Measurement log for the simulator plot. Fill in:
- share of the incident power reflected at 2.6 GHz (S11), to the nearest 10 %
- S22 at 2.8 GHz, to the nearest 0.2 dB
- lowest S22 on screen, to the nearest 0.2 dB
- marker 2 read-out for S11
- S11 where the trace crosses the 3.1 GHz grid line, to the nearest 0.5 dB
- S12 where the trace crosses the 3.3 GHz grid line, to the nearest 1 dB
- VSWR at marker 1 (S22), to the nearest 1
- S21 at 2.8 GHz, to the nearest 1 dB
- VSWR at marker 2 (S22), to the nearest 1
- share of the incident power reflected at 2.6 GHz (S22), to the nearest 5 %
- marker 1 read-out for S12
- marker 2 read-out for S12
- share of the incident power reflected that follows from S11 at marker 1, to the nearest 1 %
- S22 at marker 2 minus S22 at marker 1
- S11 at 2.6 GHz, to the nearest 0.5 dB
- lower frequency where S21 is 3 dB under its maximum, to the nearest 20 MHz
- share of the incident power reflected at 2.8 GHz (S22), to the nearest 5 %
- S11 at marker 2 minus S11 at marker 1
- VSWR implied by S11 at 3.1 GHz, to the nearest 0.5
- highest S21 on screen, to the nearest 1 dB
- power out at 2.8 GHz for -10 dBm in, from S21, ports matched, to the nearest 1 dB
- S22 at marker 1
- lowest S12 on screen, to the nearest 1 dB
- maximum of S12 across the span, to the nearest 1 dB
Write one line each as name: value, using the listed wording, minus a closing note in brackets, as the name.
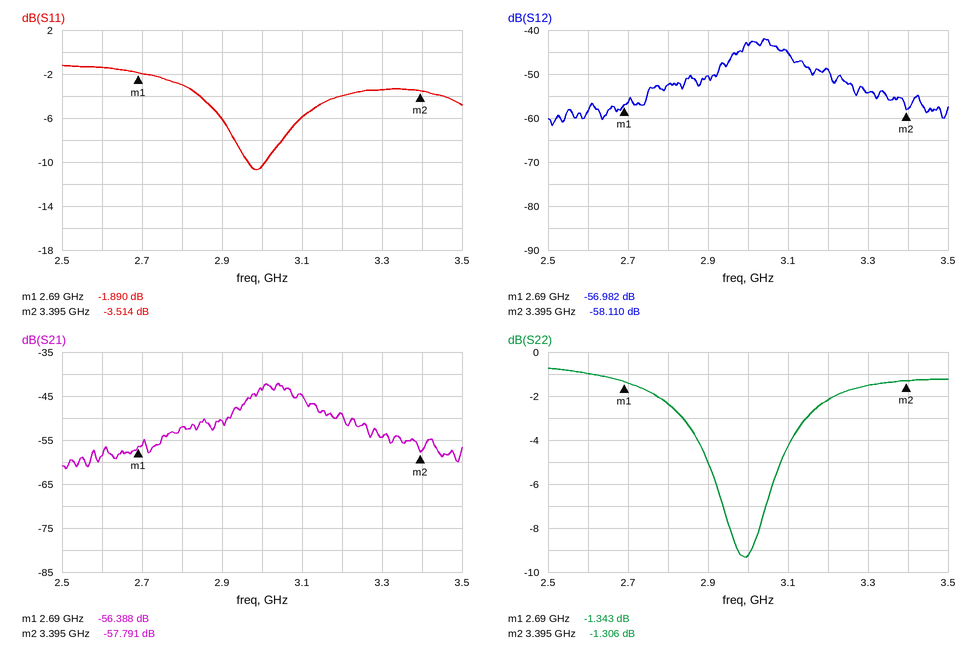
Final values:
share of the incident power reflected at 2.6 GHz (S11), to the nearest 10 %: 70 %
S22 at 2.8 GHz, to the nearest 0.2 dB: -2.4 dB
lowest S22 on screen, to the nearest 0.2 dB: -9.4 dB
marker 2 read-out for S11: -3.514 dB
S11 where the trace crosses the 3.1 GHz grid line, to the nearest 0.5 dB: -6.0 dB
S12 where the trace crosses the 3.3 GHz grid line, to the nearest 1 dB: -54 dB
VSWR at marker 1 (S22), to the nearest 1: 13
S21 at 2.8 GHz, to the nearest 1 dB: -52 dB
VSWR at marker 2 (S22), to the nearest 1: 13
share of the incident power reflected at 2.6 GHz (S22), to the nearest 5 %: 80 %
marker 1 read-out for S12: -56.982 dB
marker 2 read-out for S12: -58.110 dB
share of the incident power reflected that follows from S11 at marker 1, to the nearest 1 %: 65 %
S22 at marker 2 minus S22 at marker 1: 0.037 dB
S11 at 2.6 GHz, to the nearest 0.5 dB: -1.5 dB
lower frequency where S21 is 3 dB under its maximum, to the nearest 20 MHz: 2.98 GHz
share of the incident power reflected at 2.8 GHz (S22), to the nearest 5 %: 60 %
S11 at marker 2 minus S11 at marker 1: -1.624 dB
VSWR implied by S11 at 3.1 GHz, to the nearest 0.5: 3.0
highest S21 on screen, to the nearest 1 dB: -42 dB
power out at 2.8 GHz for -10 dBm in, from S21, ports matched, to the nearest 1 dB: -62 dBm
S22 at marker 1: -1.343 dB
lowest S12 on screen, to the nearest 1 dB: -62 dB
maximum of S12 across the span, to the nearest 1 dB: -42 dB
